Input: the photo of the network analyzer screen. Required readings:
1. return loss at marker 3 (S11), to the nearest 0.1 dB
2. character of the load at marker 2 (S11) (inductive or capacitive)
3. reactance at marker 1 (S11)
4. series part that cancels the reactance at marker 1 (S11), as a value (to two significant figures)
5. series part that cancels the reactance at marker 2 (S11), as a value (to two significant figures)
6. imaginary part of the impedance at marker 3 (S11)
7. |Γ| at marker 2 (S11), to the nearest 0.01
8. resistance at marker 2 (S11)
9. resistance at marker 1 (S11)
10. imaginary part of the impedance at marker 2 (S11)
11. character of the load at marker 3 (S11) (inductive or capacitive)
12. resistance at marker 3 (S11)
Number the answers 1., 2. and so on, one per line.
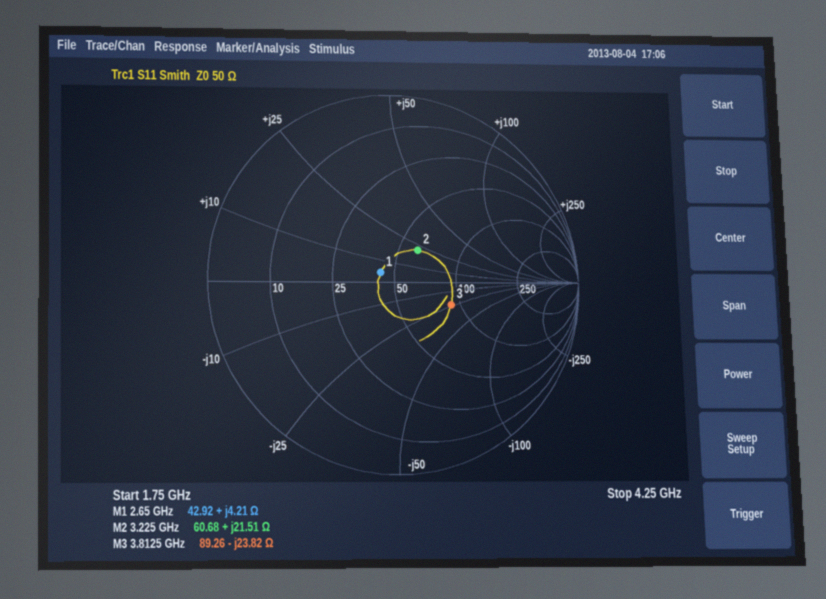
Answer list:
1. 9.8 dB
2. inductive
3. +4.21 Ω
4. 14 pF
5. 2.3 pF
6. -23.82 Ω
7. 0.21
8. 60.68 Ω
9. 42.92 Ω
10. +21.51 Ω
11. capacitive
12. 89.26 Ω
